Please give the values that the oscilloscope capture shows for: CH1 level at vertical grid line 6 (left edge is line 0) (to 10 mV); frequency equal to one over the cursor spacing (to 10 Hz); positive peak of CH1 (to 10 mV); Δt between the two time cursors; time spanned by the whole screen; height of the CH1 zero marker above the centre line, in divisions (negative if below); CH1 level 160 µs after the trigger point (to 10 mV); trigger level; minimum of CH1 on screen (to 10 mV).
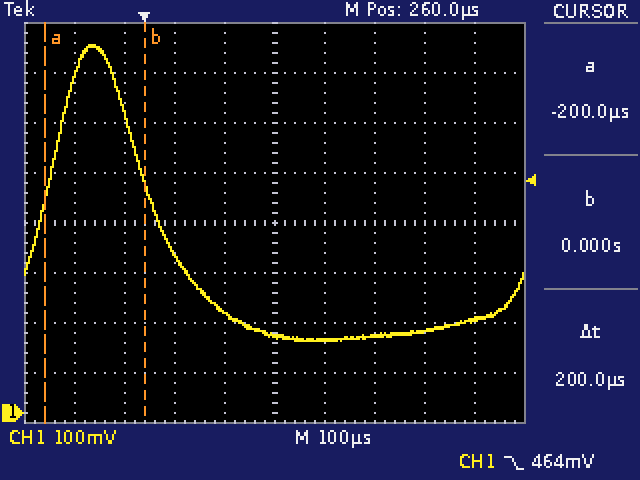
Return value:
150 mV
5.00 kHz
740 mV
200 µs
1 ms
-3.8 div
200 mV
464 mV
140 mV
